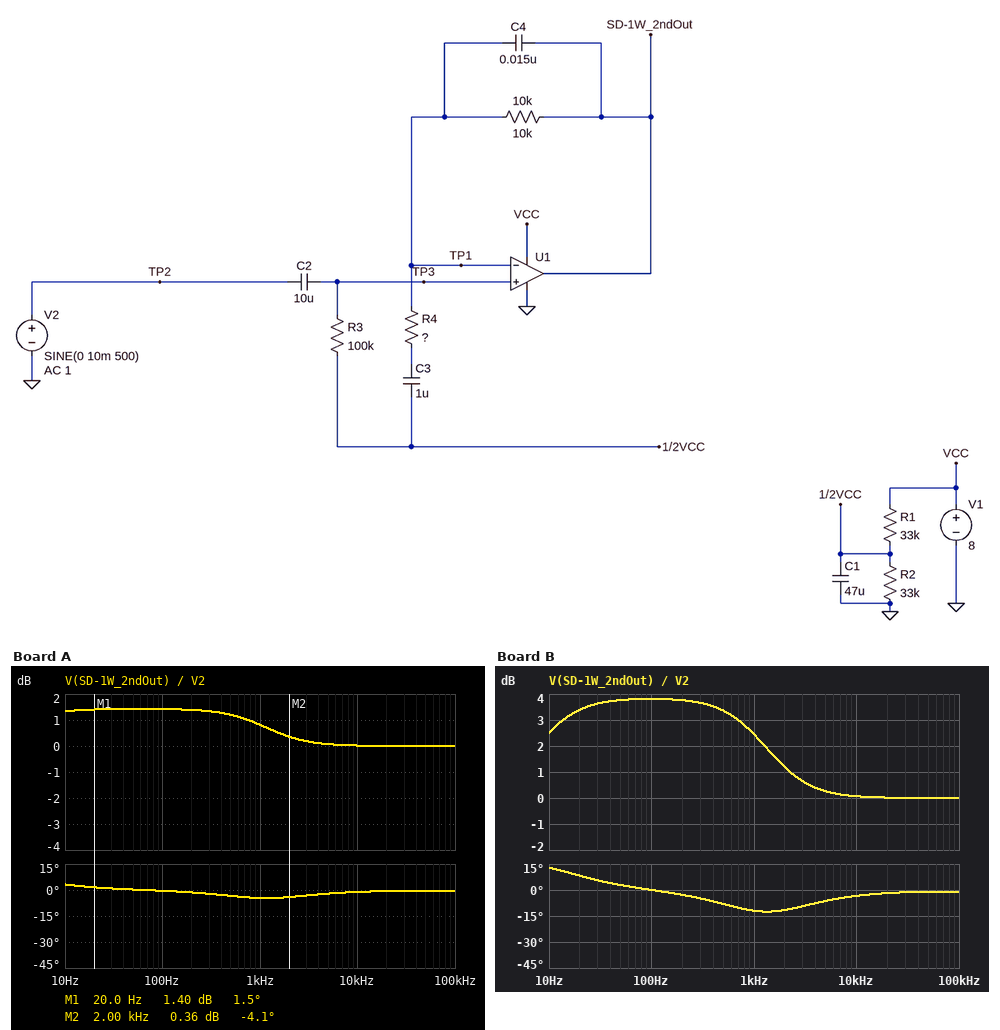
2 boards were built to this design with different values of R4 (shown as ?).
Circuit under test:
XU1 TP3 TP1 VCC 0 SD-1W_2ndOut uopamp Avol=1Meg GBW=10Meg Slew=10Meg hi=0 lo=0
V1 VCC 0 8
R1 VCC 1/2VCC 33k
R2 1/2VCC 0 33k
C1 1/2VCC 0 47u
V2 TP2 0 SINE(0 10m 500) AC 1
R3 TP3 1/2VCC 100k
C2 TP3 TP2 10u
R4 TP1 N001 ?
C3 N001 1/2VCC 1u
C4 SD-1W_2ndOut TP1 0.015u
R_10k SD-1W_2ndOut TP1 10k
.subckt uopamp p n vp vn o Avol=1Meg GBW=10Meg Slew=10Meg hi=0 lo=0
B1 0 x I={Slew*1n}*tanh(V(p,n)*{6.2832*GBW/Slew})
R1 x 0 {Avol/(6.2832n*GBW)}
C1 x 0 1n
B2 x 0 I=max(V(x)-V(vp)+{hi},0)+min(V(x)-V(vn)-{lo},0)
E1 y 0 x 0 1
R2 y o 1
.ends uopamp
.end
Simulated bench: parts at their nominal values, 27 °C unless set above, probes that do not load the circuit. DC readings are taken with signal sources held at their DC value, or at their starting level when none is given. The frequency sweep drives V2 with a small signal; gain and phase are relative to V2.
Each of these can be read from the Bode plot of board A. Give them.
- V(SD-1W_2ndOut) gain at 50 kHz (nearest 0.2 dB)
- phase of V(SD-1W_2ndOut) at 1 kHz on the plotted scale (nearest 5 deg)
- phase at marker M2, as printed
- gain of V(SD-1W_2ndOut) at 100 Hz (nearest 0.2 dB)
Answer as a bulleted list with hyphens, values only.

- 0 dB
- -5 deg
- -4.1 deg
- 1.4 dB
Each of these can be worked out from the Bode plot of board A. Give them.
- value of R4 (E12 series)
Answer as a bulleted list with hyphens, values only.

- 56 kΩ
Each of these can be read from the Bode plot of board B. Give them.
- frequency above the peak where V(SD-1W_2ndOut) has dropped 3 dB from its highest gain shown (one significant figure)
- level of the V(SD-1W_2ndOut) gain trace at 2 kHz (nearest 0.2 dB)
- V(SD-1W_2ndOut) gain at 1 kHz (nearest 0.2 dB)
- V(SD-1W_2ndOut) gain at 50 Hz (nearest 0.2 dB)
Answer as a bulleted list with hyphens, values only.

- 3 kHz
- 1.2 dB
- 2.4 dB
- 3.8 dB
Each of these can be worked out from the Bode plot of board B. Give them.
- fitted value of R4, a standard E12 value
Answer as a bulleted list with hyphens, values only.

- 18 kΩ
